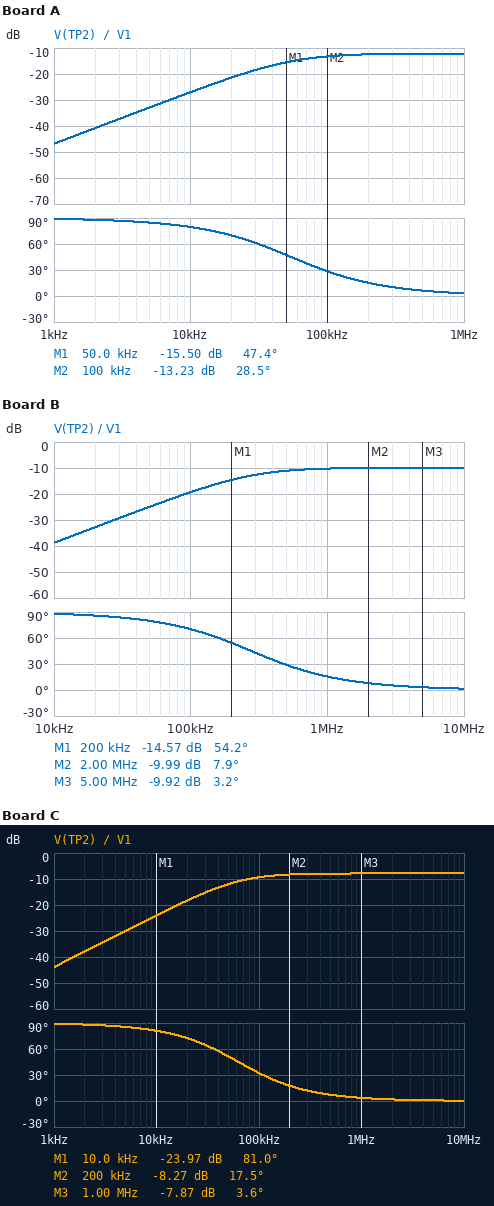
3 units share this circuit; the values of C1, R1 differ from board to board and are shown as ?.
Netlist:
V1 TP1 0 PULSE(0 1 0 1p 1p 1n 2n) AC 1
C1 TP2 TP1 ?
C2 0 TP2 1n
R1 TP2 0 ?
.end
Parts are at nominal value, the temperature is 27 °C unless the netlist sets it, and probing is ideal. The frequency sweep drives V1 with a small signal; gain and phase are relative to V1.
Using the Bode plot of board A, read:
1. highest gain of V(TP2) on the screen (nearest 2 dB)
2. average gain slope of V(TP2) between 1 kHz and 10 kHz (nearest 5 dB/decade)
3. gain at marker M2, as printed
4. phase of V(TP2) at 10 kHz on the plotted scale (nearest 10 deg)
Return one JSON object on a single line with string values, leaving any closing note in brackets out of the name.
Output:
{"highest gain of V(TP2) on the screen": "-12 dB", "average gain slope of V(TP2) between 1 kHz and 10 kHz": "20 dB/decade", "gain at marker M2, as printed": "-13.23 dB", "phase of V(TP2) at 10 kHz on the plotted scale": "80 deg"}
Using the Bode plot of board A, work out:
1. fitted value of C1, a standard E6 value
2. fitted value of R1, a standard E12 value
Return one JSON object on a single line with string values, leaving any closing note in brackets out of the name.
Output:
{"fitted value of C1, a standard E6 value": "330 pF", "fitted value of R1, a standard E12 value": "2.2 kΩ"}
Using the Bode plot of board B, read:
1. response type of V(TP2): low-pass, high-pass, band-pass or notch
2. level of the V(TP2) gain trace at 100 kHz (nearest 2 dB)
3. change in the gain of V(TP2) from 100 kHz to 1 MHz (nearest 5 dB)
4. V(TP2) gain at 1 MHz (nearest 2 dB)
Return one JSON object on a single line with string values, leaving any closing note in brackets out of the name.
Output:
{"response type of V(TP2): low-pass, high-pass, band-pass or notch": "high-pass", "level of the V(TP2) gain trace at 100 kHz": "-20 dB", "change in the gain of V(TP2) from 100 kHz to 1 MHz": "10 dB", "V(TP2) gain at 1 MHz": "-10 dB"}
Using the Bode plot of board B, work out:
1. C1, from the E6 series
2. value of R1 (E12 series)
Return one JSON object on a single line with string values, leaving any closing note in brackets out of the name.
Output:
{"C1, from the E6 series": "470 pF", "value of R1": "390 Ω"}
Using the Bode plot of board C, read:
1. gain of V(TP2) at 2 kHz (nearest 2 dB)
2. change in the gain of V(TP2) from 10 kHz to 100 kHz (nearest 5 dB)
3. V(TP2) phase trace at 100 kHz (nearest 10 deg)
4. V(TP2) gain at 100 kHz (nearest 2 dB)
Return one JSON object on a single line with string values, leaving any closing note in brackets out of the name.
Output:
{"gain of V(TP2) at 2 kHz": "-38 dB", "change in the gain of V(TP2) from 10 kHz to 100 kHz": "15 dB", "V(TP2) phase trace at 100 kHz": "30 deg", "V(TP2) gain at 100 kHz": "-10 dB"}
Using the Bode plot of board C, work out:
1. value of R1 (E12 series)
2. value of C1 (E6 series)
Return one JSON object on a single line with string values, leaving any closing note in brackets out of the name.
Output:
{"value of R1": "1.5 kΩ", "value of C1": "680 pF"}
